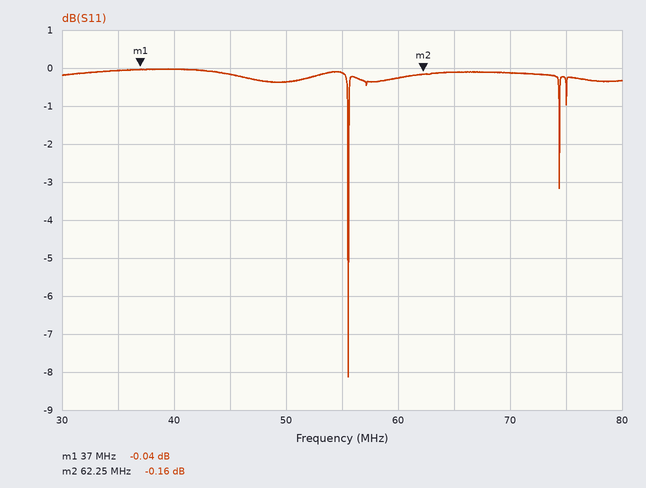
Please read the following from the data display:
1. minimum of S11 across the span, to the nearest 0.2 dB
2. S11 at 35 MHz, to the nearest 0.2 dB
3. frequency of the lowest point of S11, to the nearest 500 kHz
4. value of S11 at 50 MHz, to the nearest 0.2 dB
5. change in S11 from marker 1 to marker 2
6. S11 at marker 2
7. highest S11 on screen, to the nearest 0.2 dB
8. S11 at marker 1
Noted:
-8.2 dB
0.0 dB
55.5 MHz
-0.4 dB
-0.12 dB
-0.16 dB
0.0 dB
-0.04 dB
